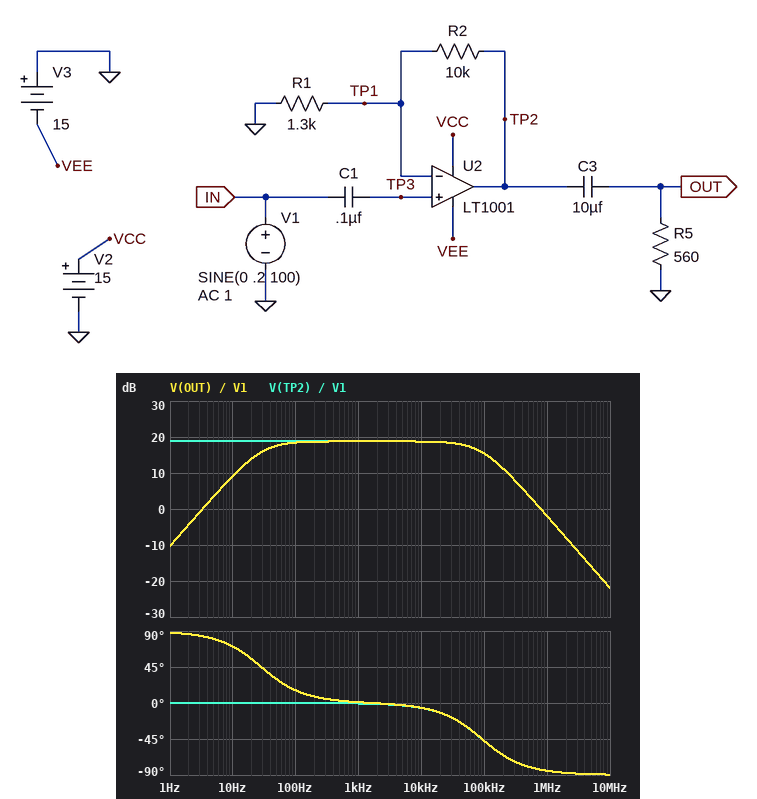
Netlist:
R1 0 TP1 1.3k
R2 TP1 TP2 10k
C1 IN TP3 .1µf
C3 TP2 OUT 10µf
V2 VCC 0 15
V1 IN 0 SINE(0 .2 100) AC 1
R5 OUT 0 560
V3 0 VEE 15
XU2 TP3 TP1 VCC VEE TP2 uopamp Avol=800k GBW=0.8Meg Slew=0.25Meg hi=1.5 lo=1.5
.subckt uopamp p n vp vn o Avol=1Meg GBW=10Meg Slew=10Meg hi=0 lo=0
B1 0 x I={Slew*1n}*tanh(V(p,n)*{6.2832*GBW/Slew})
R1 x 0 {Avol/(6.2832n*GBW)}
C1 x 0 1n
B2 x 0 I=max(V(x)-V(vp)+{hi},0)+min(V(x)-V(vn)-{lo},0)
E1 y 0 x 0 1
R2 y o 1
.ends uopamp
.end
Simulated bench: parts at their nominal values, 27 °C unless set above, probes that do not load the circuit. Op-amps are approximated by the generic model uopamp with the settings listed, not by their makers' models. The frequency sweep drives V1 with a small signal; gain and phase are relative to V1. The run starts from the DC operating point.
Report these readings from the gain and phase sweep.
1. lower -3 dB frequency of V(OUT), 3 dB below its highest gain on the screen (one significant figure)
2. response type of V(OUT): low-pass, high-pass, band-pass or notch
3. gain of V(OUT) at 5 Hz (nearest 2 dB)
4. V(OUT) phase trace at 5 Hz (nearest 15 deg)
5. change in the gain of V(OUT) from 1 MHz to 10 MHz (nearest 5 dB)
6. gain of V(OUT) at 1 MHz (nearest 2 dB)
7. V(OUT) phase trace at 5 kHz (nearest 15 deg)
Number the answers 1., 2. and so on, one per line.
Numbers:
1. 30 Hz
2. band-pass
3. 4 dB
4. 75 deg
5. -20 dB
6. -2 dB
7. 0 deg
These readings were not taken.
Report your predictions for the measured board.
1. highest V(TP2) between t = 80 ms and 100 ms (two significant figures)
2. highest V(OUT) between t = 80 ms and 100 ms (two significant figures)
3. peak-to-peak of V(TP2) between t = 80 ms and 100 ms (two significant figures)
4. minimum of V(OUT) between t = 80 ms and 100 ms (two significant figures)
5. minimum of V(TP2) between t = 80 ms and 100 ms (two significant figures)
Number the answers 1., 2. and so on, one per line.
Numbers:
1. 1.7 V
2. 1.7 V
3. 3.5 V
4. -1.7 V
5. -1.7 V
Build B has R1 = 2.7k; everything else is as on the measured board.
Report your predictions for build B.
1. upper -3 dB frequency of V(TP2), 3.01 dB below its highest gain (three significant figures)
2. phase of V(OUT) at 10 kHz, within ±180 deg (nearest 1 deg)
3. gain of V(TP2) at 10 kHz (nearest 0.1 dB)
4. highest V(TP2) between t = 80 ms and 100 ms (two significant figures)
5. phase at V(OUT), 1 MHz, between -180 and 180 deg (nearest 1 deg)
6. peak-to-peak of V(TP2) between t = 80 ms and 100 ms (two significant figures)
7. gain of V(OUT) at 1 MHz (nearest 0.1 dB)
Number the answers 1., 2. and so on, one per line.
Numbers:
1. 170 kHz
2. -3 deg
3. 13.4 dB
4. 940 mV
5. -80 deg
6. 1.9 V
7. -2.1 dB
